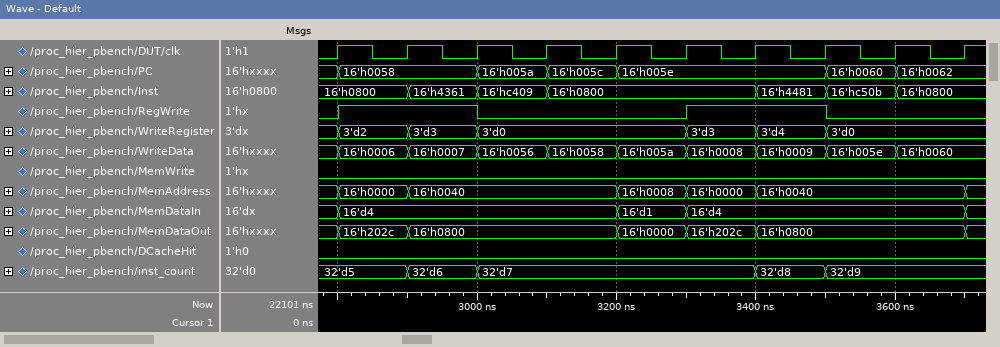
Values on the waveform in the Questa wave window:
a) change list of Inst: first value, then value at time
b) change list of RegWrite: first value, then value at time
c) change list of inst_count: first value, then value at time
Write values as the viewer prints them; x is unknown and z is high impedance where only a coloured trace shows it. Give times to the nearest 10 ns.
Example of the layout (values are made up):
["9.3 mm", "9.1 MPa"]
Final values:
["16'h0800, 16'h4361 at 2900 ns, 16'hc409 at 3000 ns, 16'h0800 at 3100 ns, 16'h4481 at 3400 ns, 16'hc50b at 3500 ns, 16'h0800 at 3600 ns", "0, 1 at 2800 ns, 0 at 3000 ns, 1 at 3300 ns, 0 at 3500 ns", "32'd5, 32'd6 at 2900 ns, 32'd7 at 3000 ns, 32'd8 at 3400 ns, 32'd9 at 3500 ns"]
